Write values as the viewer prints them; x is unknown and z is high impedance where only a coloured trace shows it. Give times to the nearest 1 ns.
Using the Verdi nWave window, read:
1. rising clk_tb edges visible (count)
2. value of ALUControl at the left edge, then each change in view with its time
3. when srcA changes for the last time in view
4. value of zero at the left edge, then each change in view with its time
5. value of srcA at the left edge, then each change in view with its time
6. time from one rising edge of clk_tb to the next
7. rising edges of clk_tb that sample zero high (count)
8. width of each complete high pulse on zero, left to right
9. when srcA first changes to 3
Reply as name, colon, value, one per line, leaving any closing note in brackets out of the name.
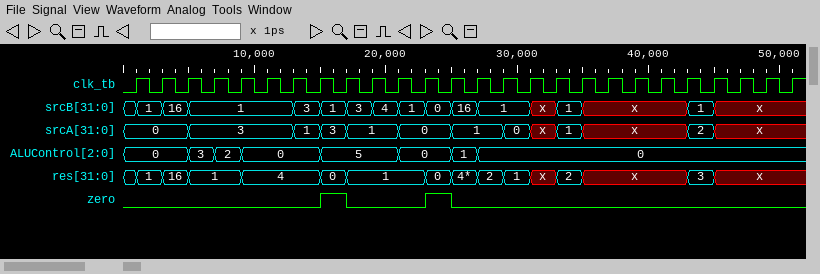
rising clk_tb edges visible: 26
value of ALUControl at the left edge, then each change in view with its time: 0, 3 at 5 ns, 2 at 7 ns, 0 at 9 ns, 5 at 15 ns, 0 at 21 ns, 1 at 25 ns, 0 at 27 ns
when srcA changes for the last time in view: 45 ns
value of zero at the left edge, then each change in view with its time: 0, 1 at 15 ns, 0 at 17 ns, 1 at 23 ns, 0 at 25 ns
value of srcA at the left edge, then each change in view with its time: 0, 3 at 5 ns, 1 at 13 ns, 3 at 15 ns, 1 at 17 ns, 0 at 21 ns, 1 at 25 ns, 0 at 29 ns, x at 31 ns, 1 at 33 ns, x at 35 ns, 2 at 43 ns, x at 45 ns
time from one rising edge of clk_tb to the next: 2 ns
rising edges of clk_tb that sample zero high: 2
width of each complete high pulse on zero, left to right: 2 ns, 2 ns
when srcA first changes to 3: 5 ns
